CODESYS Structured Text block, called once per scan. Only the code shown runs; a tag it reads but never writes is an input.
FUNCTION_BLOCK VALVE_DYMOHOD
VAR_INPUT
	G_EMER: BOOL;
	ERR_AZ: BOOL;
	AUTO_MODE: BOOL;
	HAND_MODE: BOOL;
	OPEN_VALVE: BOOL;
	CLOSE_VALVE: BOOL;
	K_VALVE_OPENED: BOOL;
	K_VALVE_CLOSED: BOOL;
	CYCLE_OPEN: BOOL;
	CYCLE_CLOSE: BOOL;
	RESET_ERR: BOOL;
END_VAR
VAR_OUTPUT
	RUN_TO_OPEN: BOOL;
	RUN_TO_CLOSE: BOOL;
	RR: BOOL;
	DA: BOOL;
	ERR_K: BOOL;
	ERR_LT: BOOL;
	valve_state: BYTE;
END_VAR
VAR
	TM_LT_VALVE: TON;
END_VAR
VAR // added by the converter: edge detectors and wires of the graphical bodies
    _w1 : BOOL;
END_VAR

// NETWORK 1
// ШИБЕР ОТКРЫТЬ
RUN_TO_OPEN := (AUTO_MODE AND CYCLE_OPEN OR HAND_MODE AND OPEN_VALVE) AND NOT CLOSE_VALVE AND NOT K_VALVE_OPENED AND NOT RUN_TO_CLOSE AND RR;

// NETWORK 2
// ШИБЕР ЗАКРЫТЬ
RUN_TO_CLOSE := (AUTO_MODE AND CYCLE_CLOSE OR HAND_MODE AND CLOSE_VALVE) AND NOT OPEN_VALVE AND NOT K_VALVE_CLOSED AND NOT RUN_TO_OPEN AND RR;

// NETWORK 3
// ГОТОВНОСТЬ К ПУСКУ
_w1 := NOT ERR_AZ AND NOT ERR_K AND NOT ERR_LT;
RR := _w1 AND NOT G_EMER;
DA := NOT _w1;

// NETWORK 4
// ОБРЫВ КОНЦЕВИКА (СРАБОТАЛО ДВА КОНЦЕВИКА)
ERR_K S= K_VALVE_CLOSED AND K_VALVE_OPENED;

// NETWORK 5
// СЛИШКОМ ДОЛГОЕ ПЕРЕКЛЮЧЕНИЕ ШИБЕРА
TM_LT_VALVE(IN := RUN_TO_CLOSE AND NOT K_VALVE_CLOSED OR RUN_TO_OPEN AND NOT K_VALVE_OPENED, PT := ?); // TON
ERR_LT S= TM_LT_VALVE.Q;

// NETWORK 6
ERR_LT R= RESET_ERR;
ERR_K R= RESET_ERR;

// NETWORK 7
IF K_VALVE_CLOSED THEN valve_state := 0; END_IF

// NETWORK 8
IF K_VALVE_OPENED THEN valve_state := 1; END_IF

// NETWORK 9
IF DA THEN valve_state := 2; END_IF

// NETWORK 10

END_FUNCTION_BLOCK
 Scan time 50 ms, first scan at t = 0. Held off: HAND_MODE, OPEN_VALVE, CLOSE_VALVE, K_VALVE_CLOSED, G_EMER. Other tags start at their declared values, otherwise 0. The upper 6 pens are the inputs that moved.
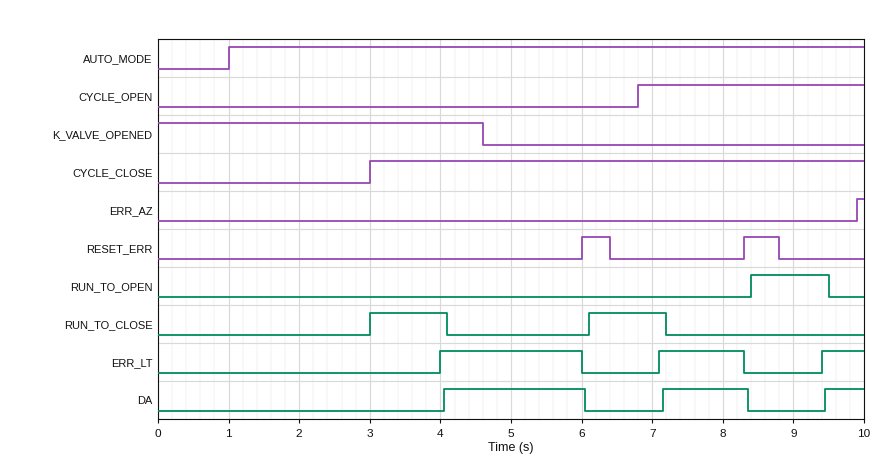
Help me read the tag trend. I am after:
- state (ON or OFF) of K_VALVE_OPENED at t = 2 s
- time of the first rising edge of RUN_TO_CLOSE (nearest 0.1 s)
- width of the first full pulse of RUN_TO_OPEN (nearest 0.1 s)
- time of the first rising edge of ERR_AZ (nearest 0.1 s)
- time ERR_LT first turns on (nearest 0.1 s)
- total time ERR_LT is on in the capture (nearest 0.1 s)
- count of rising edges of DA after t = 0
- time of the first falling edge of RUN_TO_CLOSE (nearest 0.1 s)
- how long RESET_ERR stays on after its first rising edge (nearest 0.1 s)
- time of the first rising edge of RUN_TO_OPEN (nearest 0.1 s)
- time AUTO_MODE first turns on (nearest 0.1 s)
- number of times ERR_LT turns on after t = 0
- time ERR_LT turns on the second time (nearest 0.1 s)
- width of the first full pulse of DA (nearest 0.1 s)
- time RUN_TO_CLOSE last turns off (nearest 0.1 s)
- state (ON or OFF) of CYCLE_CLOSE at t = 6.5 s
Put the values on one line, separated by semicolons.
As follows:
ON; 3.0 s; 1.1 s; 9.9 s; 4.0 s; 3.8 s; 3; 4.1 s; 0.4 s; 8.4 s; 1.0 s; 3; 7.1 s; 2.0 s; 7.2 s; ON
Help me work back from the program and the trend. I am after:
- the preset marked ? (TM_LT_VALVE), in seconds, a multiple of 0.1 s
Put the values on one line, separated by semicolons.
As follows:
1.0 s
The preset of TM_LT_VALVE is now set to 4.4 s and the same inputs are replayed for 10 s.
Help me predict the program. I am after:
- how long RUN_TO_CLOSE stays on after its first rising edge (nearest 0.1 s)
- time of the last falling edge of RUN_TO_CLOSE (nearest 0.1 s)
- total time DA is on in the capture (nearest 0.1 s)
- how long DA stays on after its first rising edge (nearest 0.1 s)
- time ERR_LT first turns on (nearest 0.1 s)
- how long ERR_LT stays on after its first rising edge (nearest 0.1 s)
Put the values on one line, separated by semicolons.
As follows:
4.5 s; 7.5 s; 1.0 s; 0.9 s; 7.4 s; 0.9 s
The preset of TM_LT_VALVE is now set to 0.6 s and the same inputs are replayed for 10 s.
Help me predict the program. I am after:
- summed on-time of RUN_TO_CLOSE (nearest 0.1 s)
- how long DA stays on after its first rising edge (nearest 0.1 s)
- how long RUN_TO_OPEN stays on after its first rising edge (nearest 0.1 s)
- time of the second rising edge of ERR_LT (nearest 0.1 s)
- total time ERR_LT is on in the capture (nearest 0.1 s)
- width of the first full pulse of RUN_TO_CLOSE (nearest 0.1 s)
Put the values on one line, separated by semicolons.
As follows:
1.4 s; 2.4 s; 0.7 s; 6.7 s; 5.0 s; 0.7 s
